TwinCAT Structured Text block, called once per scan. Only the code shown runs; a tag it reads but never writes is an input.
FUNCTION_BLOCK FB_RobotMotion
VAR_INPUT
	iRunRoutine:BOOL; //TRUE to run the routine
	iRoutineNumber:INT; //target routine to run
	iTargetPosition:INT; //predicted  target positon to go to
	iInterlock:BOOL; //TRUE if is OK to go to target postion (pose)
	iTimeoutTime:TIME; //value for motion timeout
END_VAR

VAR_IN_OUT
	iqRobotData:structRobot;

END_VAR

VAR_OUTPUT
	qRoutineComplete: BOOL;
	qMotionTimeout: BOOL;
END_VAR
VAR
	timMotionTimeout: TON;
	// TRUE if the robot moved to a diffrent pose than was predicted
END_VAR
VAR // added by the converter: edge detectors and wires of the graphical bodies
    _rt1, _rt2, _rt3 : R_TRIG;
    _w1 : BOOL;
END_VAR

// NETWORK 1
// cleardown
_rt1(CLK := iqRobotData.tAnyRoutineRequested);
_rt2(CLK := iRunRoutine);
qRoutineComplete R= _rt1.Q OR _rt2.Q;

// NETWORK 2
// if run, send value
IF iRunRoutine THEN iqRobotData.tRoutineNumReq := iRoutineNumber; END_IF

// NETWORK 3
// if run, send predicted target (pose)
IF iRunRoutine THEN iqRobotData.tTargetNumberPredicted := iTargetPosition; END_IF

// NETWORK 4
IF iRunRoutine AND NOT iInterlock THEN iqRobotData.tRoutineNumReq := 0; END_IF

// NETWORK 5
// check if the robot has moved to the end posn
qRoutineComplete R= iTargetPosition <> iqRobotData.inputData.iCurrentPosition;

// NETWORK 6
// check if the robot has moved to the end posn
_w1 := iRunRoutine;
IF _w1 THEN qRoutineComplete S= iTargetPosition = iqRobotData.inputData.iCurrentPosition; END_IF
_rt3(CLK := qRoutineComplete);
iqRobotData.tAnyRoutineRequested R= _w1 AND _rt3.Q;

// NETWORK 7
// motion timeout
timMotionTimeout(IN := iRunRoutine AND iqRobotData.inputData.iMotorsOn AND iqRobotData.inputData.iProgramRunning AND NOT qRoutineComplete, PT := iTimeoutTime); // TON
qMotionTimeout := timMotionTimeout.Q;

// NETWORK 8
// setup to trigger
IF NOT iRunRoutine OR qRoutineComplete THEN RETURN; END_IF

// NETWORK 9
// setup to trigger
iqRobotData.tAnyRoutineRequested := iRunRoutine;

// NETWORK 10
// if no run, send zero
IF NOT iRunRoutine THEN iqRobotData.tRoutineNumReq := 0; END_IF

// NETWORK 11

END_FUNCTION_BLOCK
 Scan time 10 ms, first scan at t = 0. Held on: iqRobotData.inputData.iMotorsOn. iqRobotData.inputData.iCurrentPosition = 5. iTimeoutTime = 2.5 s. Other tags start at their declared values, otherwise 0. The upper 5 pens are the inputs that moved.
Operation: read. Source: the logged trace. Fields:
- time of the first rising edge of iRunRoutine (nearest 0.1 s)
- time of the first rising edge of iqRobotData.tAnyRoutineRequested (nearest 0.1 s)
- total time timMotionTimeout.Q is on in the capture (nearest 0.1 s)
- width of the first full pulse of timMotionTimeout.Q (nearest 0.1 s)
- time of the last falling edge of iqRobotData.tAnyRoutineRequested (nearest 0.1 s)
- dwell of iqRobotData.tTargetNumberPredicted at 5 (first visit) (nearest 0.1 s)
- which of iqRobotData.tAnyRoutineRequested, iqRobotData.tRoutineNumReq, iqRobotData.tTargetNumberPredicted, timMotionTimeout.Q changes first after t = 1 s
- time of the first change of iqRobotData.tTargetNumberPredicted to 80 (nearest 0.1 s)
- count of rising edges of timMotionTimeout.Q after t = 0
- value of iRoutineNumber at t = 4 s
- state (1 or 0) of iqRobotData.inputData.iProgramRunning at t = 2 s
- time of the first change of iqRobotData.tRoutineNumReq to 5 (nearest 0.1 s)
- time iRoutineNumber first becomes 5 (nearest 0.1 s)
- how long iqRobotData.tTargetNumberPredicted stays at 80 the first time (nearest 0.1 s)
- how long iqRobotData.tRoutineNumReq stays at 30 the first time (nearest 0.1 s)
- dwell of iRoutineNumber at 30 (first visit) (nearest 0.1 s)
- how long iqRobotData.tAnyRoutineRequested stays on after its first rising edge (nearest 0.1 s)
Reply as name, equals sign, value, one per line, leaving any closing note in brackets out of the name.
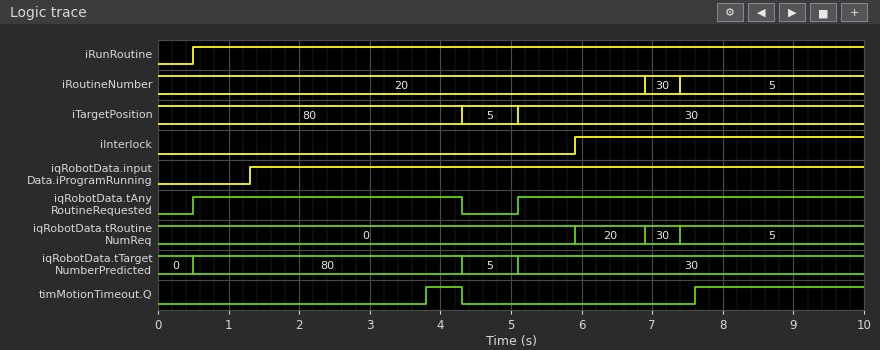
time of the first rising edge of iRunRoutine = 0.5 s
time of the first rising edge of iqRobotData.tAnyRoutineRequested = 0.5 s
total time timMotionTimeout.Q is on in the capture = 2.9 s
width of the first full pulse of timMotionTimeout.Q = 0.5 s
time of the last falling edge of iqRobotData.tAnyRoutineRequested = 4.3 s
dwell of iqRobotData.tTargetNumberPredicted at 5 (first visit) = 0.8 s
which of iqRobotData.tAnyRoutineRequested, iqRobotData.tRoutineNumReq, iqRobotData.tTargetNumberPredicted, timMotionTimeout.Q changes first after t = 1 s = timMotionTimeout.Q
time of the first change of iqRobotData.tTargetNumberPredicted to 80 = 0.5 s
count of rising edges of timMotionTimeout.Q after t = 0 = 2
value of iRoutineNumber at t = 4 s = 20
state (1 or 0) of iqRobotData.inputData.iProgramRunning at t = 2 s = 1
time of the first change of iqRobotData.tRoutineNumReq to 5 = 7.4 s
time iRoutineNumber first becomes 5 = 7.4 s
how long iqRobotData.tTargetNumberPredicted stays at 80 the first time = 3.8 s
how long iqRobotData.tRoutineNumReq stays at 30 the first time = 0.5 s
dwell of iRoutineNumber at 30 (first visit) = 0.5 s
how long iqRobotData.tAnyRoutineRequested stays on after its first rising edge = 3.8 s
